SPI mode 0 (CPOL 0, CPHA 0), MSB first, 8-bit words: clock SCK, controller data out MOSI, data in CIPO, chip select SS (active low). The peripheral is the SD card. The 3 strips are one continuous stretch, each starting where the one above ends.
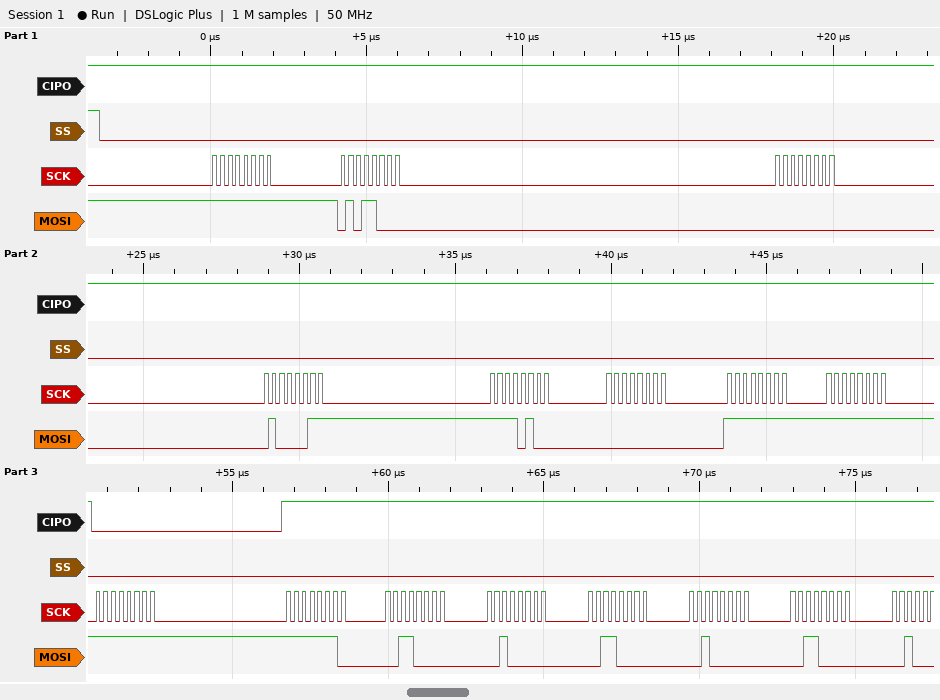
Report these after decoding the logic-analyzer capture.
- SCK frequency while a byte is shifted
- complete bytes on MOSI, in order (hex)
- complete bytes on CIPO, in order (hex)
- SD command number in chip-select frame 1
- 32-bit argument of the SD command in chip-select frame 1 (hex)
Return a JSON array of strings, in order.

["4 MHz", "FF 58 00 43 F4 00 FF FF FF FE 30 20 30 20 30", "FF FF FF FF FF FF FF FF 00 FF FF FF FF FF FF", "CMD24", "0x0043F400"]
